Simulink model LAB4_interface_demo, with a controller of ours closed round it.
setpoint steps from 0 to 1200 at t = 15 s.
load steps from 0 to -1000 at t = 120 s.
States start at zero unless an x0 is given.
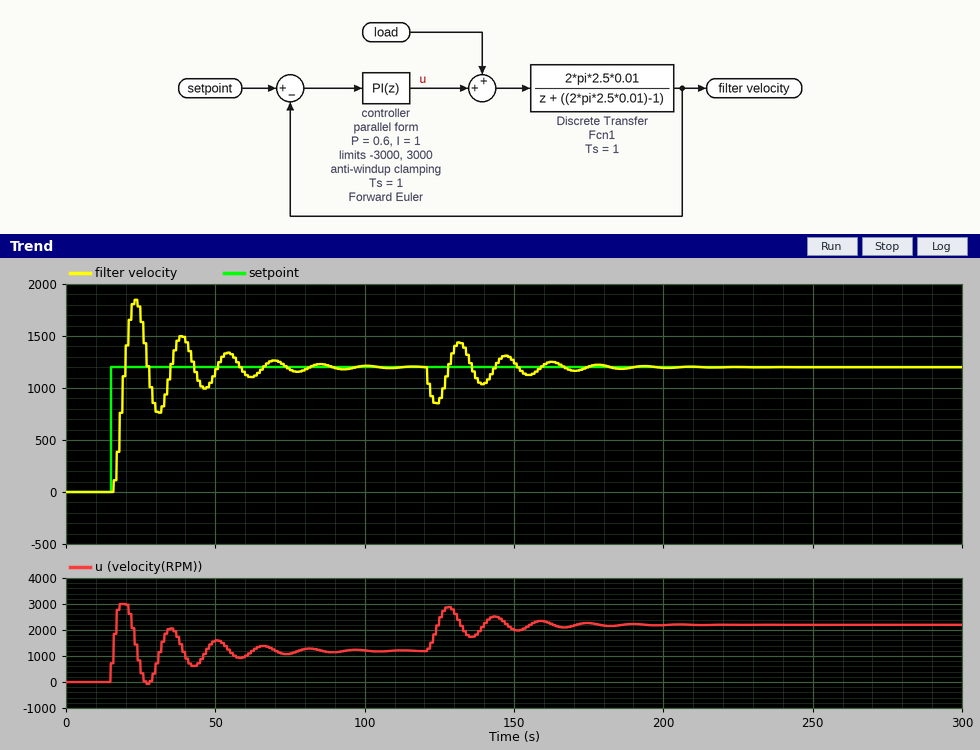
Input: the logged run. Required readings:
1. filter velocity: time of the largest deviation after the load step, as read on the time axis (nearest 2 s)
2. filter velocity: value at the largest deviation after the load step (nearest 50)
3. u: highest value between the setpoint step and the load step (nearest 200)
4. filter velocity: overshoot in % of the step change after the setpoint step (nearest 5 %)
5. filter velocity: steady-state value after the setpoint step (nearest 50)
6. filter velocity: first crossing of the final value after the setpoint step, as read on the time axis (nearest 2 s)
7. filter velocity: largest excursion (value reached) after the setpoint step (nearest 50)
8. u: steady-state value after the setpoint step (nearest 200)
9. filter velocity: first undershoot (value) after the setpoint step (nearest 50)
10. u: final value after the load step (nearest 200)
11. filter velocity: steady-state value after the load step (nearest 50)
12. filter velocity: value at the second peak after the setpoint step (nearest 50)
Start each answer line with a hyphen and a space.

- 124 s
- 850
- 3000
- 55 %
- 1200
- 20 s
- 1850
- 1200
- 750
- 2200
- 1200
- 1500
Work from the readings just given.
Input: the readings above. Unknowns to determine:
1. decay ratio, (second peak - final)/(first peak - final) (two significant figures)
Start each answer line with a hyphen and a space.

- 0.46
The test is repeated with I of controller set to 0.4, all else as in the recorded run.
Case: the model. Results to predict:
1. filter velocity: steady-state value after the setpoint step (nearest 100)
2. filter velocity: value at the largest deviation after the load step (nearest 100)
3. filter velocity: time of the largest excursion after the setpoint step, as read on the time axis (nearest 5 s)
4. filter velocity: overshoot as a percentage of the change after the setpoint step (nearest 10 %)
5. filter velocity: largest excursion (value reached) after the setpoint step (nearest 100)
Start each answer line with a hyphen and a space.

- 1200
- 800
- 25 s
- 30 %
- 1500
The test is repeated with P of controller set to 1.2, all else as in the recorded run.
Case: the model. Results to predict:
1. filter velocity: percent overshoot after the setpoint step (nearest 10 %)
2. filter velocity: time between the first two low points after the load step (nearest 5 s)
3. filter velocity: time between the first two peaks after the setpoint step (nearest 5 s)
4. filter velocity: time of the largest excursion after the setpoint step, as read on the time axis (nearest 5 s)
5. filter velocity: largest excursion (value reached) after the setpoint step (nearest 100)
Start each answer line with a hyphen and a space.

- 40 %
- 15 s
- 15 s
- 20 s
- 1700
